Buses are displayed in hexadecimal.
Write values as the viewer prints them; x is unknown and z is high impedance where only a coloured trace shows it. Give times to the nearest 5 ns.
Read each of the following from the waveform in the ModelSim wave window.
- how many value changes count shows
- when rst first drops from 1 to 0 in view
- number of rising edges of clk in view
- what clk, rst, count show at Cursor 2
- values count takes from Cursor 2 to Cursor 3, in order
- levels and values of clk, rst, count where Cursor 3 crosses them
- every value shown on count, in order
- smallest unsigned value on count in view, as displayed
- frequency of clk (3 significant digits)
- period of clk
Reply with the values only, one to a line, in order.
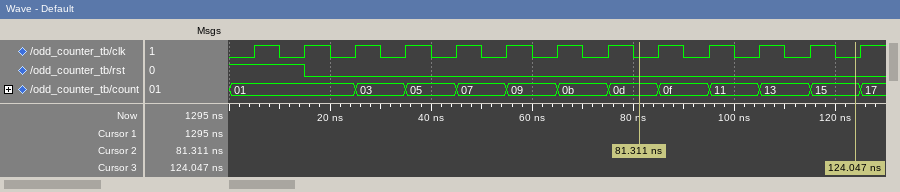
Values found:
11
15 ns
13
clk=0, rst=0, count=0d
0d, 0f, 11, 13, 15
clk=0, rst=0, count=15
01, 03, 05, 07, 09, 0b, 0d, 0f, 11, 13, 15, 17
01
100 MHz
10 ns
